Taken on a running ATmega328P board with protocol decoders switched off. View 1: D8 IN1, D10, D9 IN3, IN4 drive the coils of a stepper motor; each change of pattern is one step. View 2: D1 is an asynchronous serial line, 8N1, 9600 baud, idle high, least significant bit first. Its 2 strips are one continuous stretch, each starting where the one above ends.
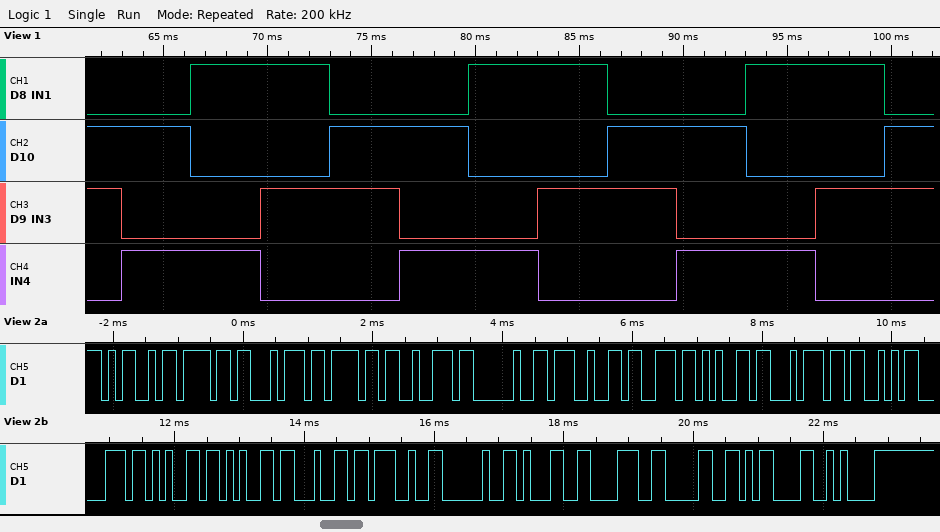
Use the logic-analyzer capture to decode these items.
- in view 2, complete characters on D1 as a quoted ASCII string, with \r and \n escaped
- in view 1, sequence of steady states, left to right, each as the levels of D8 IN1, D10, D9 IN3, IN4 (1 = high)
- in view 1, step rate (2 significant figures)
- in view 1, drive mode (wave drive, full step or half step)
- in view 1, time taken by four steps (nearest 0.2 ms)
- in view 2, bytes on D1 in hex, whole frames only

"Motor 'setSpeed' 180\r\n"
0110 0101 1001 1010 0110 0101 1001 1010 0110 0101 1001 1010 0110
300 steps/s
full step
13.4 ms
4D 6F 74 6F 72 20 27 73 65 74 53 70 65 65 64 27 20 31 38 30 0D 0A
